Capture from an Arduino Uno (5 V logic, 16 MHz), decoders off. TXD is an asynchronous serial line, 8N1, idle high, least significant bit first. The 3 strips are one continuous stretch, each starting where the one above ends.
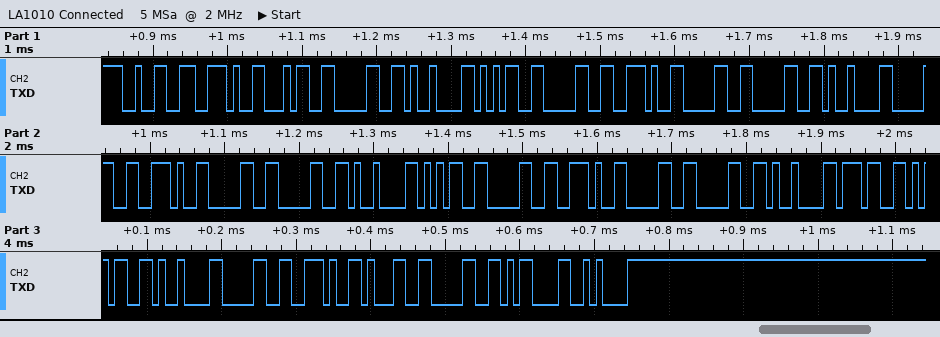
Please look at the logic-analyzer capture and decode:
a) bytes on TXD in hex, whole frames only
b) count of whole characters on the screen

32 2E 34 30 09 35 30 2E 30 30 09 30 2E 30 30 09 35 30 2E 30 30 09 37 35 09 30 2E 31 30 0D 0A
31
